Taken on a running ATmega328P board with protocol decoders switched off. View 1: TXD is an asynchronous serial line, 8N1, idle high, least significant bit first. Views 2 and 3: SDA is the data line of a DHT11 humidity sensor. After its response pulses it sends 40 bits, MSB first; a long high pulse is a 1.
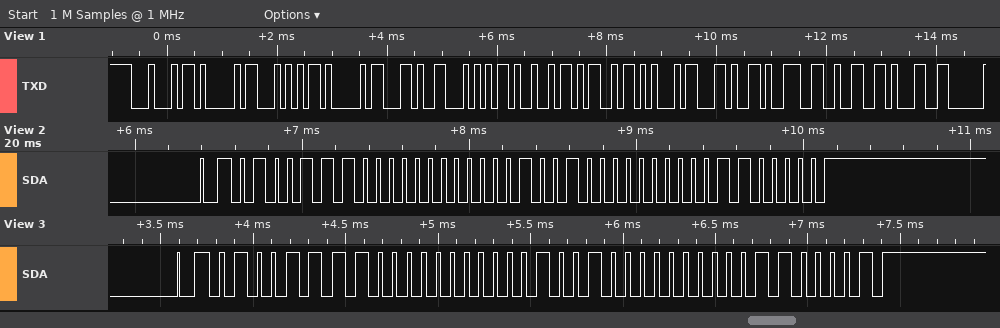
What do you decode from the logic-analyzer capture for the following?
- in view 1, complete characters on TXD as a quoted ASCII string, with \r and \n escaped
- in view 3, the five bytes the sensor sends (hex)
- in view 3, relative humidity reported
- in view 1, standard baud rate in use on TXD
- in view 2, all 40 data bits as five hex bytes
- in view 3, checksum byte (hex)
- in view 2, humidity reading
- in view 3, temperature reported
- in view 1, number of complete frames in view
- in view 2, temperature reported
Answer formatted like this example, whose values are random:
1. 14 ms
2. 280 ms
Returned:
1. "DATA,TIME,921"
2. 4F 00 12 00 61
3. 79 %
4. 9600 baud
5. 4E 00 12 00 60
6. 0x61
7. 78 %
8. 18.0 °C
9. 13
10. 18.0 °C
